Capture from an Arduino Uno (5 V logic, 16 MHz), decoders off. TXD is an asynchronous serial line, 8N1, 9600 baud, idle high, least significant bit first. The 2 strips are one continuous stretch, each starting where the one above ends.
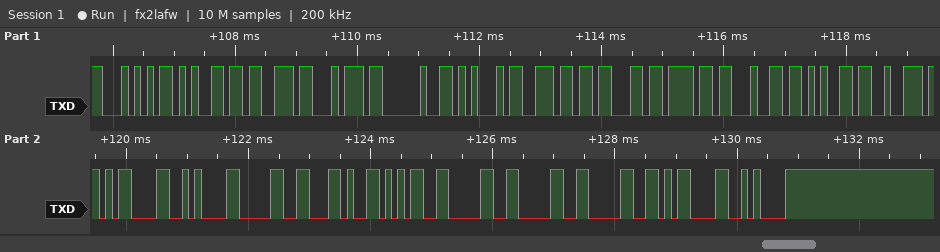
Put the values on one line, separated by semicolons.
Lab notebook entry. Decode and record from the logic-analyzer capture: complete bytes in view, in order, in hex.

0x54 0x65 0x73 0x74 0x20 0x45 0x6E 0x63 0x6F 0x64 0x65 0x72 0x0D 0x0A 0x30 0x2C 0x35 0x30 0x30 0x30 0x0D 0x0A
